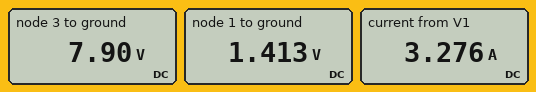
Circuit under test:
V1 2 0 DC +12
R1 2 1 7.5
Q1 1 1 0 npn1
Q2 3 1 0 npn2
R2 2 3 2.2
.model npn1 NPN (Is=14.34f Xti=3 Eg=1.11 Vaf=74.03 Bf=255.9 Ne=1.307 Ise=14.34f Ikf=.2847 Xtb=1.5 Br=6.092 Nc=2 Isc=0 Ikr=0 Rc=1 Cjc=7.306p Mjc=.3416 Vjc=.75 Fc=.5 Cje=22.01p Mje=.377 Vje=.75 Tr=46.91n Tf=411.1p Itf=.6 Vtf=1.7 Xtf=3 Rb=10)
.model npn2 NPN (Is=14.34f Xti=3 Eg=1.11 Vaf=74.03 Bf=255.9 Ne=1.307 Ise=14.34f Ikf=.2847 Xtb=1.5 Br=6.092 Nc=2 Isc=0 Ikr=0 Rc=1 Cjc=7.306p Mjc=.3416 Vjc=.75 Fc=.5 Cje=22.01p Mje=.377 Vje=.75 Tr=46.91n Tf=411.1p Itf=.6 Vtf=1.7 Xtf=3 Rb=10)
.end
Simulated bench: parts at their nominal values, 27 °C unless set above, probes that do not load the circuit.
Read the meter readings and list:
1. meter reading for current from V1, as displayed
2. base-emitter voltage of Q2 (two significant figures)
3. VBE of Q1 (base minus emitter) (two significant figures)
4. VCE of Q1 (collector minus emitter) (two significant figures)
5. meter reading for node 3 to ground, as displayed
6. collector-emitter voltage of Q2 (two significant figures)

3.276 A
1.4 V
1.4 V
1.4 V
7.90 V
7.9 V
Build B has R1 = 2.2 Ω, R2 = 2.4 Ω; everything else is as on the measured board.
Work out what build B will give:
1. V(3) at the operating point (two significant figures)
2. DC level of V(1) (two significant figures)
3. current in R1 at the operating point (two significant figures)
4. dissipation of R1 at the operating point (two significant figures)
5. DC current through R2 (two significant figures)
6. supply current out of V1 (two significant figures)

3.6 V
3.5 V
3.9 A
33 W
3.5 A
7.4 A
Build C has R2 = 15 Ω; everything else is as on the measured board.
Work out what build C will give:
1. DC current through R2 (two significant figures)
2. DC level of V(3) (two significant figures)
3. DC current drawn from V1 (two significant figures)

750 mA
810 mV
2.2 A
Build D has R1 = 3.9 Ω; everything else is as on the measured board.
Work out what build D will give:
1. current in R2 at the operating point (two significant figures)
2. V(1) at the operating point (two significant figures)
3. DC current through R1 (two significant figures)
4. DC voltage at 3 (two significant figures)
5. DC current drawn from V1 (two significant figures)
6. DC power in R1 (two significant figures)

3.0 A
2.3 V
2.5 A
5.4 V
5.5 A
24 W
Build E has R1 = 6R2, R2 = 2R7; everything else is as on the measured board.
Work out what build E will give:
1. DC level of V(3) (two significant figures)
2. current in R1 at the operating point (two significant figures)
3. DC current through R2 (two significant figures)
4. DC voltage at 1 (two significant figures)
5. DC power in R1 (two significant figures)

6.1 V
1.7 A
2.2 A
1.6 V
17 W
